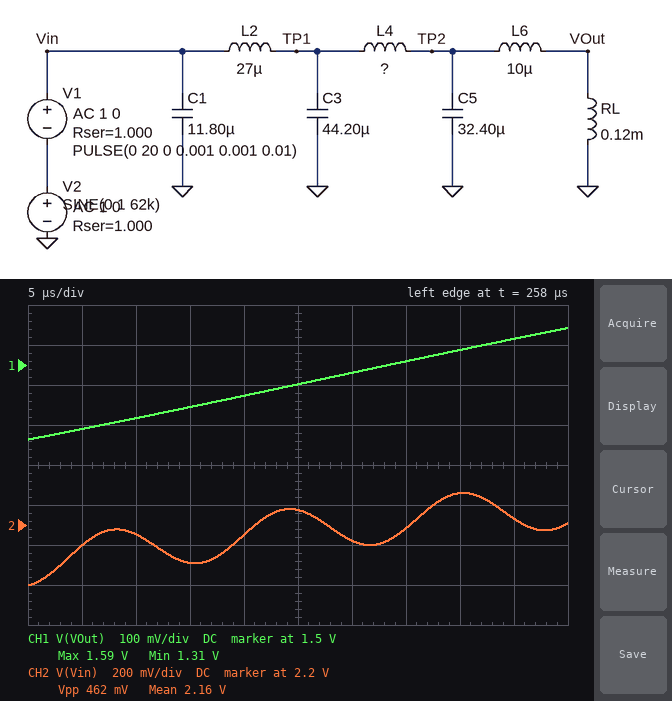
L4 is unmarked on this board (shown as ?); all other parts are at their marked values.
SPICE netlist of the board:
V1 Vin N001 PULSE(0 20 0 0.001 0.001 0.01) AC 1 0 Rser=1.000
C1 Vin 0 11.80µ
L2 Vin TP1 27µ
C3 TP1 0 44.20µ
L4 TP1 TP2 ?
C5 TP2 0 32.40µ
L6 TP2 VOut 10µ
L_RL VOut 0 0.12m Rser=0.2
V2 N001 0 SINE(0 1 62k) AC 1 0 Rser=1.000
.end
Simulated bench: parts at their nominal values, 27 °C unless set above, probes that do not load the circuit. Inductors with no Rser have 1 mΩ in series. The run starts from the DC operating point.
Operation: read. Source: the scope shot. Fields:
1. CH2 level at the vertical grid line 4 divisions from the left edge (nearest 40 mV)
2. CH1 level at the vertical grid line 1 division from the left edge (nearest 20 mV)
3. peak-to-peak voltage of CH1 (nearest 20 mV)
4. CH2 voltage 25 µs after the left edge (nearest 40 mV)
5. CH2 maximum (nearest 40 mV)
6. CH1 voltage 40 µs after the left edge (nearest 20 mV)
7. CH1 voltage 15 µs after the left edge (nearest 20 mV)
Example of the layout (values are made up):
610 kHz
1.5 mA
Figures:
2.16 V
1.34 V
280 mV
2.28 V
2.36 V
1.54 V
1.40 V
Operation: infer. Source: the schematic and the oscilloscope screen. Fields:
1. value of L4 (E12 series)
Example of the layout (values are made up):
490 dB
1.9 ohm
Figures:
39 µH
